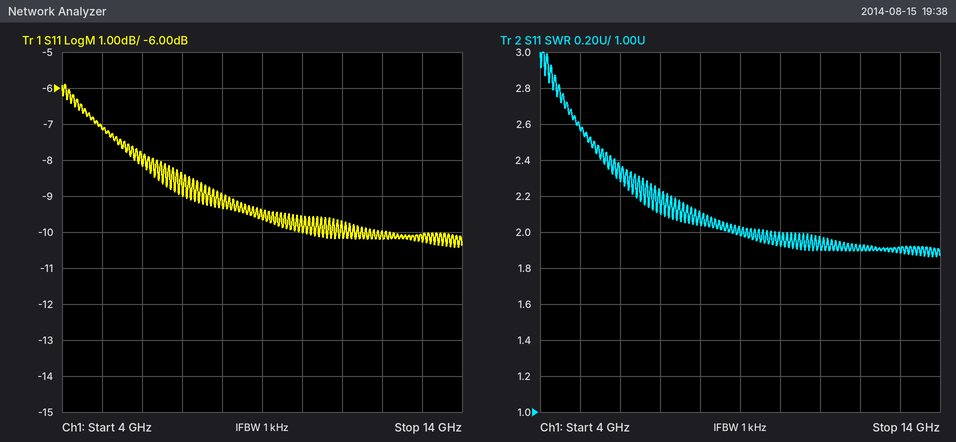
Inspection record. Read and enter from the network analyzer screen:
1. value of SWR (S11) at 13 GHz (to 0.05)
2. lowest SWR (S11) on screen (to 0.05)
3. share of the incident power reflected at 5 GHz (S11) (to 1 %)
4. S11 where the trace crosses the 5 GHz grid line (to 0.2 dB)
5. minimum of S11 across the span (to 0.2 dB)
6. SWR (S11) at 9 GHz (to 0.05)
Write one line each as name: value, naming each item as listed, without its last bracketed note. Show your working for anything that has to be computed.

value of SWR (S11) at 13 GHz: 1.90
lowest SWR (S11) on screen: 1.85
share of the incident power reflected at 5 GHz (S11): 10^(-7.2/10) ≈ 19 %
S11 where the trace crosses the 5 GHz grid line: -7.2 dB
minimum of S11 across the span: -10.4 dB
SWR (S11) at 9 GHz: 2.00
